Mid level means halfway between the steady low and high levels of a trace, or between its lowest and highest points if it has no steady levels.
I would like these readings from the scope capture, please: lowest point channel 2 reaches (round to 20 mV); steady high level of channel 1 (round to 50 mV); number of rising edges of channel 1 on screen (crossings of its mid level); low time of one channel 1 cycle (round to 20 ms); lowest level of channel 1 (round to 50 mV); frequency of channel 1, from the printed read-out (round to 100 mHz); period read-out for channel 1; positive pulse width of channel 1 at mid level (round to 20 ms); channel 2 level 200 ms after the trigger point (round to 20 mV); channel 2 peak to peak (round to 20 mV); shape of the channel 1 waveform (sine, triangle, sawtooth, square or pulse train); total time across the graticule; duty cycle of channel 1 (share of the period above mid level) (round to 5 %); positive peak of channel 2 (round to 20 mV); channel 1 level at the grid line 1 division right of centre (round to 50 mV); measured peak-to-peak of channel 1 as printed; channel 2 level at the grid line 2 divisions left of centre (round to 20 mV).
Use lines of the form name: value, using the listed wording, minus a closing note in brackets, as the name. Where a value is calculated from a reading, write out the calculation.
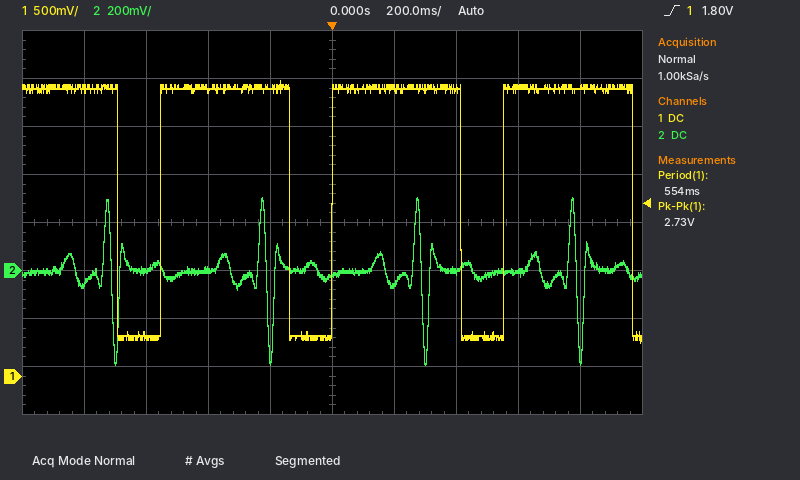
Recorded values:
lowest point channel 2 reaches: -400 mV
steady high level of channel 1: 3.00 V
number of rising edges of channel 1 on screen: 3
low time of one channel 1 cycle: 140 ms
lowest level of channel 1: 350 mV
frequency of channel 1, from the printed read-out: 1 / 554 ms ≈ 1.8 Hz
period read-out for channel 1: 554 ms
positive pulse width of channel 1 at mid level: 420 ms
channel 2 level 200 ms after the trigger point: -60 mV
channel 2 peak to peak: 300 mV − (-400 mV) = 700 mV
shape of the channel 1 waveform: pulse train
total time across the graticule: 2 s
duty cycle of channel 1 (share of the period above mid level): 75 %
positive peak of channel 2: 300 mV
channel 1 level at the grid line 1 division right of centre: 3.00 V
measured peak-to-peak of channel 1 as printed: 2.73 V
channel 2 level at the grid line 2 divisions left of centre: 0 mV
